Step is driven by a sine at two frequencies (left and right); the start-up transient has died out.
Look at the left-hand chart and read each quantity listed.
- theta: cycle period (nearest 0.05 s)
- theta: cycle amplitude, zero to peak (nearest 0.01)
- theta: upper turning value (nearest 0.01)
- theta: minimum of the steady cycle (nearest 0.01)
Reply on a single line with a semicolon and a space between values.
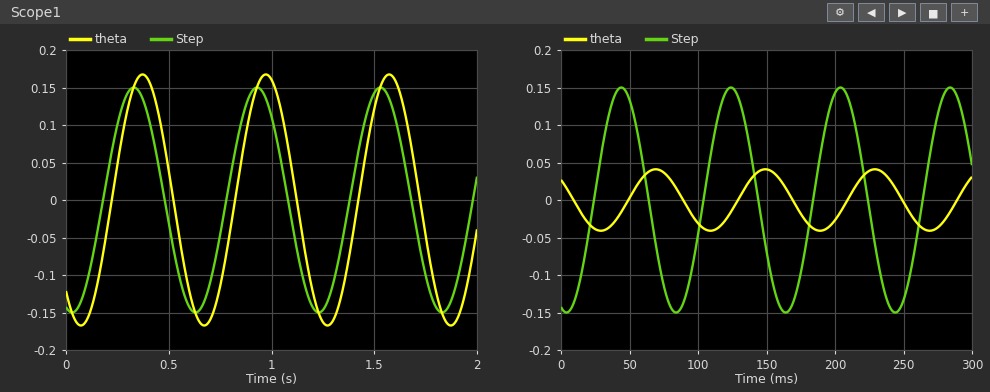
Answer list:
0.60 s; 0.17; 0.17; -0.17
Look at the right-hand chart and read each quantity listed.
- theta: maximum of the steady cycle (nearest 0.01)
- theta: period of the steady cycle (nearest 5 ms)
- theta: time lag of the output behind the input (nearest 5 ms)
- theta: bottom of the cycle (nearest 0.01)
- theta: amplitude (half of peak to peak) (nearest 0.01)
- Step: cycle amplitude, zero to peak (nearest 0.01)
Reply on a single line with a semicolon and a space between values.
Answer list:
0.04; 80 ms; 25 ms; -0.04; 0.04; 0.15
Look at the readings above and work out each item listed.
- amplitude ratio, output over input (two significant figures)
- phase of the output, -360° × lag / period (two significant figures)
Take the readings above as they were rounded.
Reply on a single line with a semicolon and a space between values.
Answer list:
0.27; -110°
